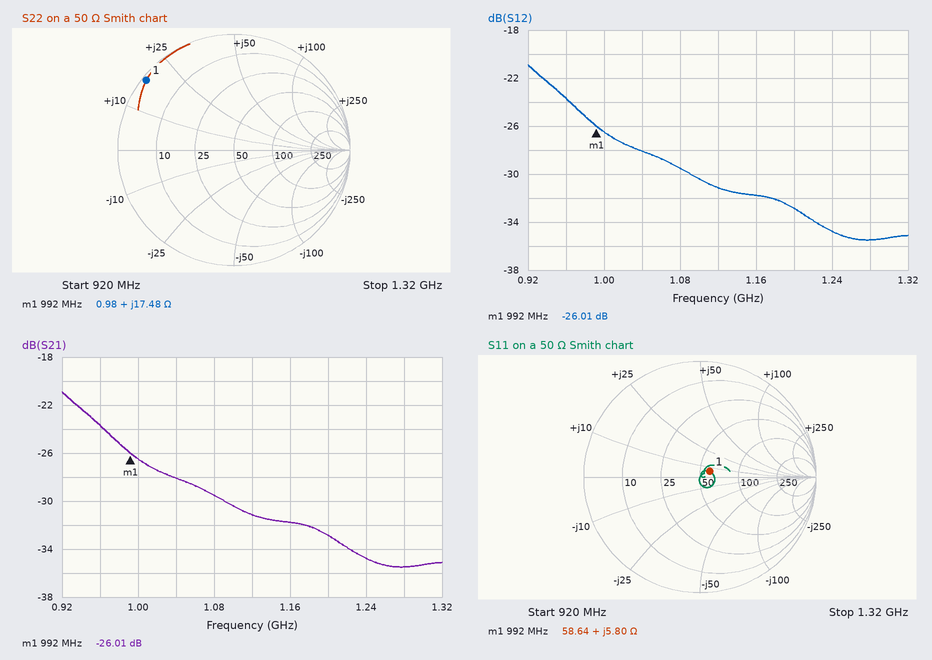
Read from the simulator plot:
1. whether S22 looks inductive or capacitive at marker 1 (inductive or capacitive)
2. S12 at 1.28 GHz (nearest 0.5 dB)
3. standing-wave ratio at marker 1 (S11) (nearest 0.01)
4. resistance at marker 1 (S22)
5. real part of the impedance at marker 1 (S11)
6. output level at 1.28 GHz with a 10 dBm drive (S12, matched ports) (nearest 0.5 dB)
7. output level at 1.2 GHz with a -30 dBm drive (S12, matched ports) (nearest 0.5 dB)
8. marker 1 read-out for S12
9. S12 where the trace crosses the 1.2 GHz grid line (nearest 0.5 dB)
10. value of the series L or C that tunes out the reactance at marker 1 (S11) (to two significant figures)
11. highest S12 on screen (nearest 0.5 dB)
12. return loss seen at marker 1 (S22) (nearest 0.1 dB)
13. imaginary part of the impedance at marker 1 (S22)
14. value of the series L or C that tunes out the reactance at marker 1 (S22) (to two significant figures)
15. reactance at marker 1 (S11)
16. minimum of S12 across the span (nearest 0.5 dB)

inductive
-35.5 dB
1.21
0.98 Ω
58.64 Ω
-25.5 dBm
-63.0 dBm
-26.01 dB
-33.0 dB
28 pF
-21.0 dB
0.3 dB
+17.48 Ω
9.2 pF
+5.80 Ω
-35.5 dB
